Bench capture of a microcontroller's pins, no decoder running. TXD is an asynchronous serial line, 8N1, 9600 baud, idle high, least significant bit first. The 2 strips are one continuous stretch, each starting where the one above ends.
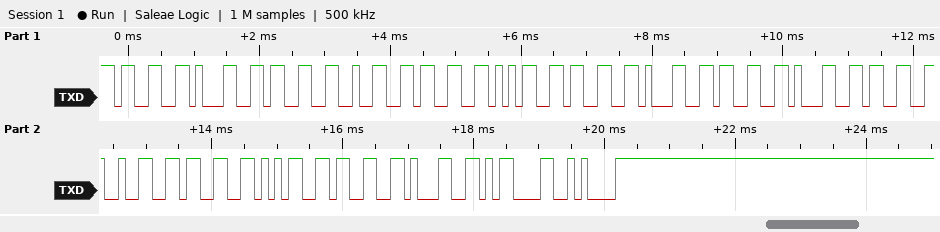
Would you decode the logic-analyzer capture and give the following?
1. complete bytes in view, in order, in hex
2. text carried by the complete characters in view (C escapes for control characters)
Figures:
33 31 33 32 33 35 33 31 33 31 33 32 33 35 33 31 0D 0A
"3132353131323531\r\n"
